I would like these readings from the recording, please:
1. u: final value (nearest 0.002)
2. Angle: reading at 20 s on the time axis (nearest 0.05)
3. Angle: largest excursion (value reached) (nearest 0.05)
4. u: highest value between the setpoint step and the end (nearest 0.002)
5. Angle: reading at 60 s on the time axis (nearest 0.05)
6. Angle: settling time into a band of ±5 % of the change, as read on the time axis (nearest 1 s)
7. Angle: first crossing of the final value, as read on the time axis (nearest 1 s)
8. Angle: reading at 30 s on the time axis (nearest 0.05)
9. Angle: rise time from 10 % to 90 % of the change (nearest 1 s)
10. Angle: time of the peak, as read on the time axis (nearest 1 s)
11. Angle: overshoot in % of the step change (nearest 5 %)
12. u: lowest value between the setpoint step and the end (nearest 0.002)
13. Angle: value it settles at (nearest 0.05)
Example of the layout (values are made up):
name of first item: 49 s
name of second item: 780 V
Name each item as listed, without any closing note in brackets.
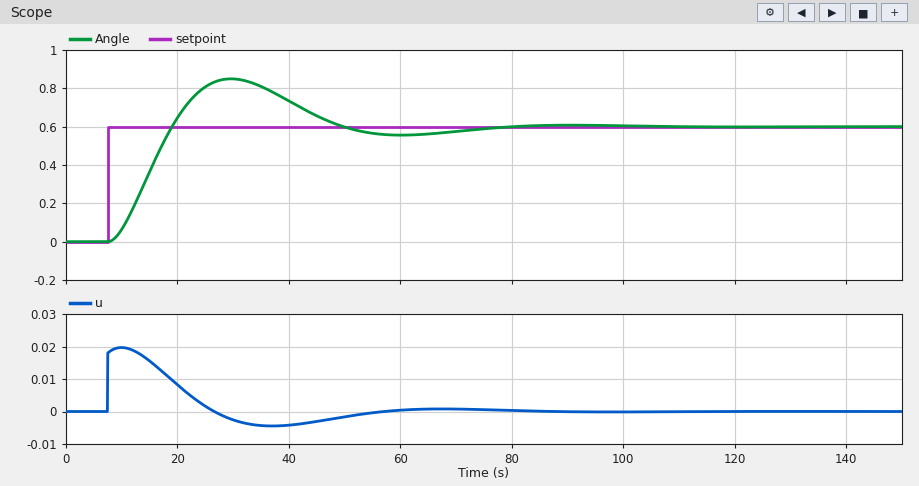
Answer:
u: final value: 0.000
Angle: reading at 20 s on the time axis: 0.65
Angle: largest excursion (value reached): 0.85
u: highest value between the setpoint step and the end: 0.020
Angle: reading at 60 s on the time axis: 0.55
Angle: settling time into a band of ±5 % of the change, as read on the time axis: 68 s
Angle: first crossing of the final value, as read on the time axis: 19 s
Angle: reading at 30 s on the time axis: 0.85
Angle: rise time from 10 % to 90 % of the change: 8 s
Angle: time of the peak, as read on the time axis: 30 s
Angle: overshoot in % of the step change: 40 %
u: lowest value between the setpoint step and the end: -0.004
Angle: value it settles at: 0.60
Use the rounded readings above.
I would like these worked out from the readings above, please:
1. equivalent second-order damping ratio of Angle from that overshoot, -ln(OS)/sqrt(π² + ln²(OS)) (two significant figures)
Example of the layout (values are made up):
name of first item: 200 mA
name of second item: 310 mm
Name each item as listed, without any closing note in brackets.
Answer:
equivalent second-order damping ratio of Angle from that overshoot, -ln(OS)/sqrt(π² + ln²(OS)): 0.28
